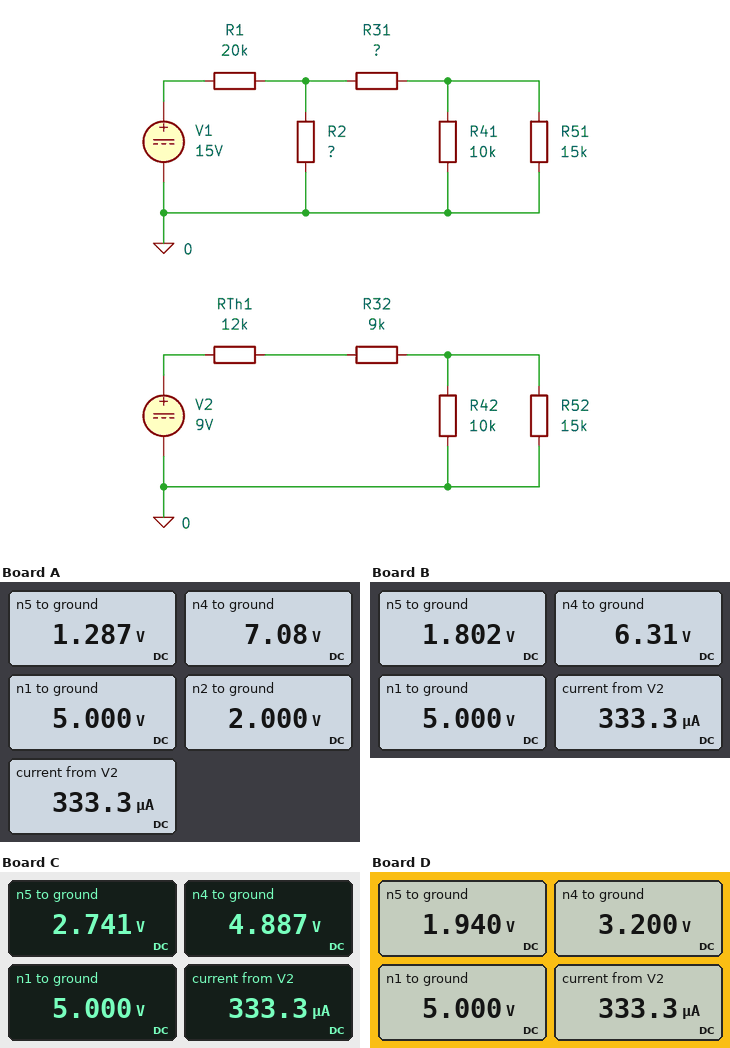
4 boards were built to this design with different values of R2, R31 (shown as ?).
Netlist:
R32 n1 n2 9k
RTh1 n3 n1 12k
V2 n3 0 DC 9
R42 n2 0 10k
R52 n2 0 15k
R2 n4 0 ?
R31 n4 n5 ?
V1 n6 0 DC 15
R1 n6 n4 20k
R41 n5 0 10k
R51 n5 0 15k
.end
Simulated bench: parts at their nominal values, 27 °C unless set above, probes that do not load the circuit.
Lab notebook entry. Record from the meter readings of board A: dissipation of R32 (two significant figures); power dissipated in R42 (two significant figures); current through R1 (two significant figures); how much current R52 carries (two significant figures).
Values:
1.0 mW
400 µW
400 µA
130 µA
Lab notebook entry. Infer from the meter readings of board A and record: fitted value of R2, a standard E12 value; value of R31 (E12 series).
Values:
39 kΩ
27 kΩ
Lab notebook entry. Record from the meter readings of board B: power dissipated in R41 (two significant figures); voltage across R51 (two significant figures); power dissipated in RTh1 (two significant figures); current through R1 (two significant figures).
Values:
320 µW
1.8 V
1.3 mW
430 µA
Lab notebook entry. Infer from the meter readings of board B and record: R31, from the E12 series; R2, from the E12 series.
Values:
15 kΩ
47 kΩ
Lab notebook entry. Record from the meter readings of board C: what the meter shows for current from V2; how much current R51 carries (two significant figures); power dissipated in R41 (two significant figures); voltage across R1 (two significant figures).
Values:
333.3 µA
180 µA
750 µW
10 V
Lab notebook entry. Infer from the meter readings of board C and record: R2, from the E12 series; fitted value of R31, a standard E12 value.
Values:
100 kΩ
4.7 kΩ
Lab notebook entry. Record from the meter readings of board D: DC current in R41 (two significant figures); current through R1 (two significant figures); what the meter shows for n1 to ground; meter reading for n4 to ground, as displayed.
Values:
190 µA
590 µA
5.000 V
3.200 V
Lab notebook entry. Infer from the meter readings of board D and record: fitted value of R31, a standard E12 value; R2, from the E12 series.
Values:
3.9 kΩ
12 kΩ
